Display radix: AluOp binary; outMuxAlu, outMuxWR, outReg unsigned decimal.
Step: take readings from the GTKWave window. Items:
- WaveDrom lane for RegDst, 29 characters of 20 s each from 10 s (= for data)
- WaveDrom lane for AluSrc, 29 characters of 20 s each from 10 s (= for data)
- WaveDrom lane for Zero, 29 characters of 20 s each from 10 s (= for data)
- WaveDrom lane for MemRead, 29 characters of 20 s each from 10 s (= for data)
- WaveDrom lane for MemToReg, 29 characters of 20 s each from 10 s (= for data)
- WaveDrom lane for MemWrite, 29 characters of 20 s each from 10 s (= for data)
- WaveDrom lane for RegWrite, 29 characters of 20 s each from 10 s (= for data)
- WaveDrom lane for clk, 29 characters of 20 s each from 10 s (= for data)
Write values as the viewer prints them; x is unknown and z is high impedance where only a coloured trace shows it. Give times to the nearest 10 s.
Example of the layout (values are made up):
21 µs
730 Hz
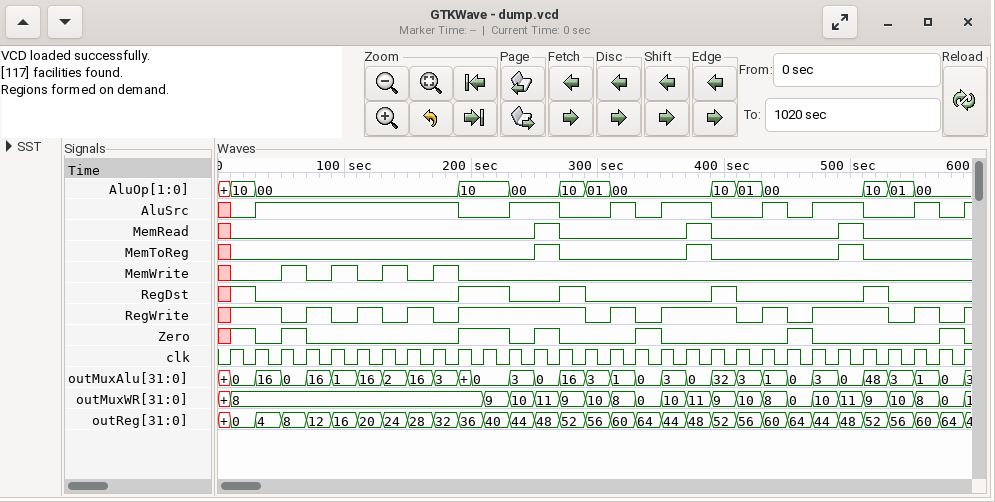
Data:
{name: 'RegDst', wave: '10.......1.0.10....10....10..'}
{name: 'AluSrc', wave: '01.......0.1.0.101.0.101.0.10'}
{name: 'Zero', wave: '1010.....1.010..10....10....1'}
{name: 'MemRead', wave: '0...........10....10....10...'}
{name: 'MemToReg', wave: '0...........10....10....10...'}
{name: 'MemWrite', wave: '0.10101010...................'}
{name: 'RegWrite', wave: '1.01010101....0101..0101..010'}
{name: 'clk', wave: 'p............................'}
